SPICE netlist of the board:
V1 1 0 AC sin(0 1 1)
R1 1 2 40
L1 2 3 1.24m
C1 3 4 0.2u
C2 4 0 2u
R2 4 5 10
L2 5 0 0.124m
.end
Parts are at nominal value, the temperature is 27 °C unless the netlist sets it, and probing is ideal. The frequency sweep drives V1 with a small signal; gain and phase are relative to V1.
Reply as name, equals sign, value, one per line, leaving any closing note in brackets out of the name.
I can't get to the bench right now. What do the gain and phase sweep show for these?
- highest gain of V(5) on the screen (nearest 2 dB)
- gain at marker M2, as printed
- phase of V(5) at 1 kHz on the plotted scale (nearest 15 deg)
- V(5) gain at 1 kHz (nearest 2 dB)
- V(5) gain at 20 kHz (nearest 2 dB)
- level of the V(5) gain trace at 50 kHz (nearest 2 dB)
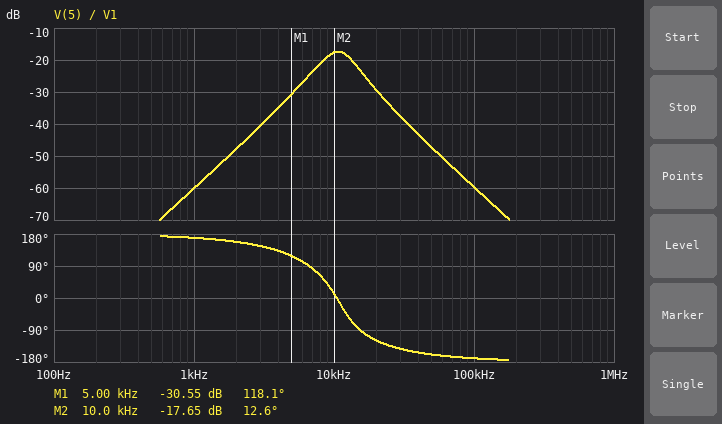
highest gain of V(5) on the screen = -18 dB
gain at marker M2, as printed = -17.65 dB
phase of V(5) at 1 kHz on the plotted scale = 165 deg
V(5) gain at 1 kHz = -60 dB
V(5) gain at 20 kHz = -30 dB
level of the V(5) gain trace at 50 kHz = -48 dB
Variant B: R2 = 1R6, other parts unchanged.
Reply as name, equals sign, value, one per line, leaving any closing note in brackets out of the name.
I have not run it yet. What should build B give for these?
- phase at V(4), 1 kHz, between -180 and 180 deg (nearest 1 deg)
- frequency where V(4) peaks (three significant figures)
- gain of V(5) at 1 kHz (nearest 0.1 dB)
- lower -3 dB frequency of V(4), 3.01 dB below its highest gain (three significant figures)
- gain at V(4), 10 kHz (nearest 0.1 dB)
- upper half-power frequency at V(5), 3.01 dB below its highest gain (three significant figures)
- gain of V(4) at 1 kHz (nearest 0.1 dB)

phase at V(4), 1 kHz, between -180 and 180 deg = 112 deg
frequency where V(4) peaks = 10.6 kHz
gain of V(5) at 1 kHz = -60.0 dB
lower -3 dB frequency of V(4), 3.01 dB below its highest gain = 8.48 kHz
gain at V(4), 10 kHz = -6.1 dB
upper half-power frequency at V(5), 3.01 dB below its highest gain = 12.4 kHz
gain of V(4) at 1 kHz = -52.8 dB
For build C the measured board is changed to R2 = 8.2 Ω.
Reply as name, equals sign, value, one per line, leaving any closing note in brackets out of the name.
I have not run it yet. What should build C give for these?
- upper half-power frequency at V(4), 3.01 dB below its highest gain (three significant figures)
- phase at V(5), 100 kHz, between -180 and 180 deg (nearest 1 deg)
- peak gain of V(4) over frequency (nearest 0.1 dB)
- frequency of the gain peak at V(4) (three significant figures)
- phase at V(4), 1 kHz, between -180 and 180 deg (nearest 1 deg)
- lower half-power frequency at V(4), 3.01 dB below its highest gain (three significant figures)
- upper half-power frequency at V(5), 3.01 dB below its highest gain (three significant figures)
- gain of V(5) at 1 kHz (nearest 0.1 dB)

upper half-power frequency at V(4), 3.01 dB below its highest gain = 13.0 kHz
phase at V(5), 100 kHz, between -180 and 180 deg = -171 deg
peak gain of V(4) over frequency = -12.9 dB
frequency of the gain peak at V(4) = 10.4 kHz
phase at V(4), 1 kHz, between -180 and 180 deg = 86 deg
lower half-power frequency at V(4), 3.01 dB below its highest gain = 7.65 kHz
upper half-power frequency at V(5), 3.01 dB below its highest gain = 13.5 kHz
gain of V(5) at 1 kHz = -60.1 dB
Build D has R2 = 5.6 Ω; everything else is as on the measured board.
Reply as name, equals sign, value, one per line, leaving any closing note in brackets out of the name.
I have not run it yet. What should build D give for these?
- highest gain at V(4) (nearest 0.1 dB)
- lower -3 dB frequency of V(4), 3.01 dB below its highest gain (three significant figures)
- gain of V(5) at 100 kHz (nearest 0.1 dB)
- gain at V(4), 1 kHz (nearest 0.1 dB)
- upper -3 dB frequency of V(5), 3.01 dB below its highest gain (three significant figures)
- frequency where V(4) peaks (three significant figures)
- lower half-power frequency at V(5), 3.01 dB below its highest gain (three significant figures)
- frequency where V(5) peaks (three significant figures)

highest gain at V(4) = -11.5 dB
lower -3 dB frequency of V(4), 3.01 dB below its highest gain = 7.95 kHz
gain of V(5) at 100 kHz = -59.7 dB
gain at V(4), 1 kHz = -42.8 dB
upper -3 dB frequency of V(5), 3.01 dB below its highest gain = 13.3 kHz
frequency where V(4) peaks = 10.5 kHz
lower half-power frequency at V(5), 3.01 dB below its highest gain = 8.32 kHz
frequency where V(5) peaks = 10.8 kHz
